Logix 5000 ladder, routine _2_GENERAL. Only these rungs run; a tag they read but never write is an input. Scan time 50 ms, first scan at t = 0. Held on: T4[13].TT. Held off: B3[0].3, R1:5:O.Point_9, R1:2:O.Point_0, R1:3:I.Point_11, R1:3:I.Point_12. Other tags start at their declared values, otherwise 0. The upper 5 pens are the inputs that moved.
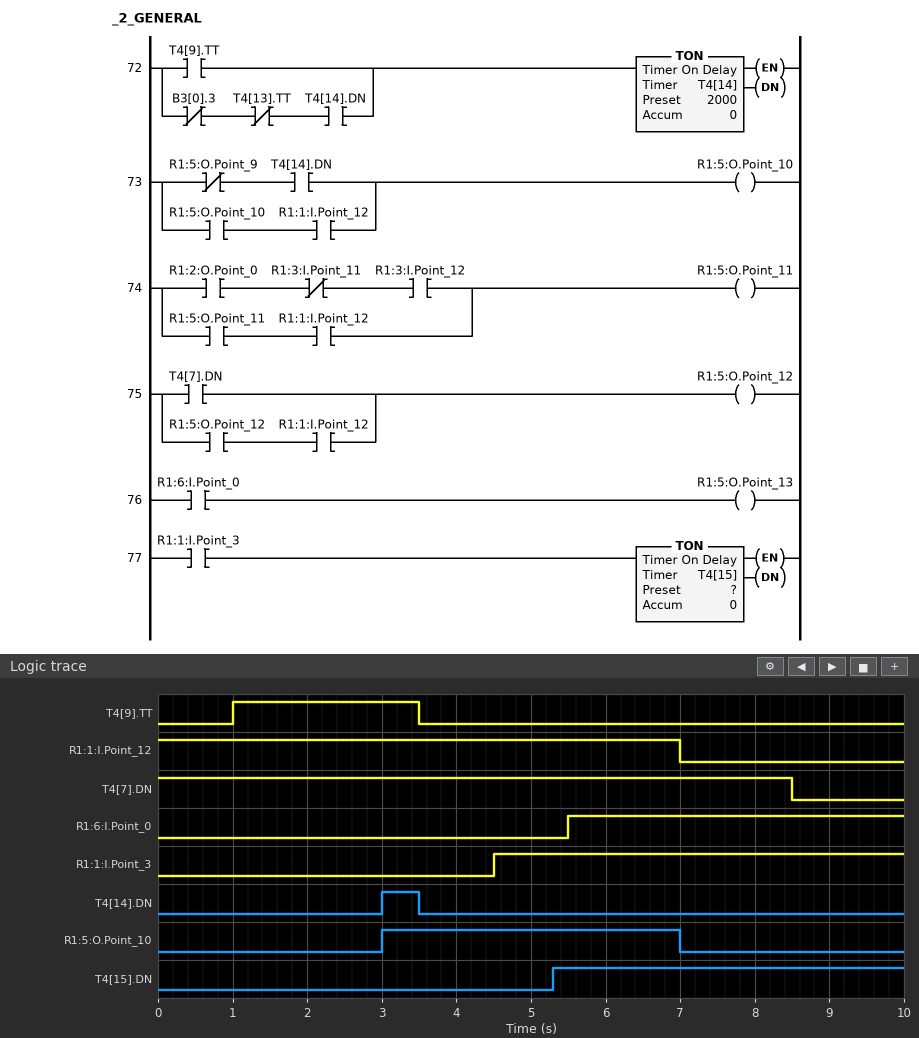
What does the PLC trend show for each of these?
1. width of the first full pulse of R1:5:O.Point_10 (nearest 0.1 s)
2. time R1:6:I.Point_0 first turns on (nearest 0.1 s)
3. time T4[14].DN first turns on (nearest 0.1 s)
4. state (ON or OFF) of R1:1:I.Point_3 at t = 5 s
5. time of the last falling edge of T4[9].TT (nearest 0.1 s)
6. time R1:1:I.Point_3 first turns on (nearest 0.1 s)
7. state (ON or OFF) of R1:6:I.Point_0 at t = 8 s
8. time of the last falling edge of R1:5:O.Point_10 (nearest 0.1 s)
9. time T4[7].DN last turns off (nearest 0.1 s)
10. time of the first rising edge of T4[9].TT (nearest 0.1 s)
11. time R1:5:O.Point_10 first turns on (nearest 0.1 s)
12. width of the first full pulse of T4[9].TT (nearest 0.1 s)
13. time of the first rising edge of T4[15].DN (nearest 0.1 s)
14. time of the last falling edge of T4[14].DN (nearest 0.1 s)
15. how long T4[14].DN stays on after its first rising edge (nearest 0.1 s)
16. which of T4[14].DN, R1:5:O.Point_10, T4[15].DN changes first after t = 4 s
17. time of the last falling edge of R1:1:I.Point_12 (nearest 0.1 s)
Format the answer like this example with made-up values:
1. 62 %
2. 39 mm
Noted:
1. 4.0 s
2. 5.5 s
3. 3.0 s
4. ON
5. 3.5 s
6. 4.5 s
7. ON
8. 7.0 s
9. 8.5 s
10. 1.0 s
11. 3.0 s
12. 2.5 s
13. 5.3 s
14. 3.5 s
15. 0.5 s
16. T4[15].DN
17. 7.0 s
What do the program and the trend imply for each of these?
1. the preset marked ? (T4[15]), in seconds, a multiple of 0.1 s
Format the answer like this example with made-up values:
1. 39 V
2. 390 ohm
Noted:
1. 0.8 s
